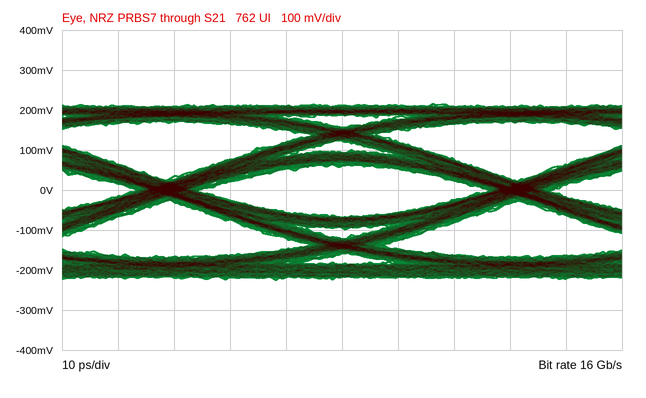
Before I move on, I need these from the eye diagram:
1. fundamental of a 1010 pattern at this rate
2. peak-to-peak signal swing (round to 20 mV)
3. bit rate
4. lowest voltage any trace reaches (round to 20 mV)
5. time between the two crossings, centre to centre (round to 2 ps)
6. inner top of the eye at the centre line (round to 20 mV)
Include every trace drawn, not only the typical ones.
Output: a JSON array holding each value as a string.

["8 GHz", "440 mV", "16 Gb/s", "-220 mV", "62 ps", "60 mV"]
